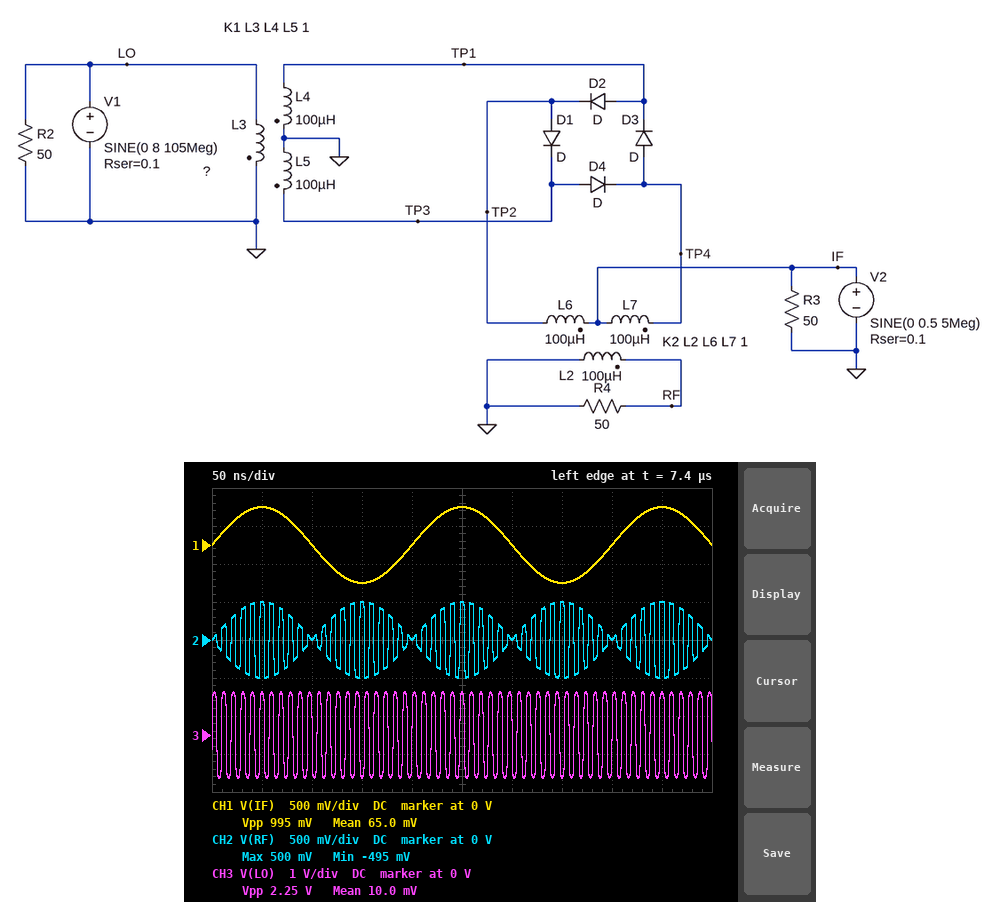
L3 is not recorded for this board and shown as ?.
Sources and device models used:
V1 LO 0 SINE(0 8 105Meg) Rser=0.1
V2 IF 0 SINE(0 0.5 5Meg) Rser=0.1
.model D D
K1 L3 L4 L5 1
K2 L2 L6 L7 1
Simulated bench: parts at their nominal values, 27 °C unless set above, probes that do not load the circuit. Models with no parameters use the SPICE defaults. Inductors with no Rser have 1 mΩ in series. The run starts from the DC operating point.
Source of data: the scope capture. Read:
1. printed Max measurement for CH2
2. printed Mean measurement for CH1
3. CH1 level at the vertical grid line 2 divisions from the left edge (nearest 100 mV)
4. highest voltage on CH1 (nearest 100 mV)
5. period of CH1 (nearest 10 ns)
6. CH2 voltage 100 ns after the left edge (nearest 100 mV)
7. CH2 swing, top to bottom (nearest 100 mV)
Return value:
500 mV
65.0 mV
0 V
500 mV
200 ns
0 V
1.0 V
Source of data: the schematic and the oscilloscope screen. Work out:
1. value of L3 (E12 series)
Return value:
120 µH
